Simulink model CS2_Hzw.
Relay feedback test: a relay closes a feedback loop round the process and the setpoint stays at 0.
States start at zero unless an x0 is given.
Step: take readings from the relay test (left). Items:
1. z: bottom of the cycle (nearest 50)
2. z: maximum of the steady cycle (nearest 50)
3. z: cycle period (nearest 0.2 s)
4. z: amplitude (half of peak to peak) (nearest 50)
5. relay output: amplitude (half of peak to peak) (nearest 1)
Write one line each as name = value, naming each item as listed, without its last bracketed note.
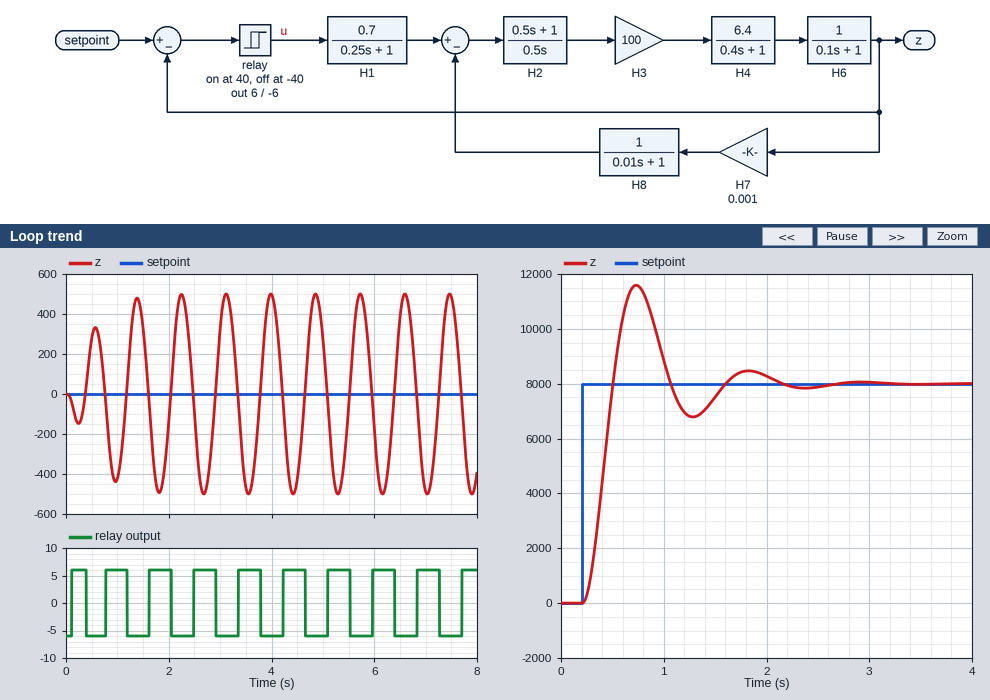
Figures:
z: bottom of the cycle = -500
z: maximum of the steady cycle = 500
z: cycle period = 0.8 s
z: amplitude (half of peak to peak) = 500
relay output: amplitude (half of peak to peak) = 6
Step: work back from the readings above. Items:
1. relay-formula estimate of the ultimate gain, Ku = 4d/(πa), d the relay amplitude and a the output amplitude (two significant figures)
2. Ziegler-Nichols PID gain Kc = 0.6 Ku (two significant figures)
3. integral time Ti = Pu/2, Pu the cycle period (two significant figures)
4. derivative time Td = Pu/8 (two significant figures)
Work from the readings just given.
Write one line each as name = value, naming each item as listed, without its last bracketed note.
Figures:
relay-formula estimate of the ultimate gain, Ku = 4d/(πa), d the relay amplitude and a the output amplitude = 0.015
Ziegler-Nichols PID gain Kc = 0.6 Ku = 0.0090
integral time Ti = Pu/2, Pu the cycle period = 0.40 s
derivative time Td = Pu/8 = 0.10 s
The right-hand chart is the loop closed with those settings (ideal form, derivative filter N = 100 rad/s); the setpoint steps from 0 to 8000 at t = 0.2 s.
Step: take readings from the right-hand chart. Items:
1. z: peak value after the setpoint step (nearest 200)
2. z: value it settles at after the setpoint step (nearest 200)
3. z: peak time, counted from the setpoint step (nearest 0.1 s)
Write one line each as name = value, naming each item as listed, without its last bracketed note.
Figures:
z: peak value after the setpoint step = 11600
z: value it settles at after the setpoint step = 8000
z: peak time, counted from the setpoint step = 0.5 s
